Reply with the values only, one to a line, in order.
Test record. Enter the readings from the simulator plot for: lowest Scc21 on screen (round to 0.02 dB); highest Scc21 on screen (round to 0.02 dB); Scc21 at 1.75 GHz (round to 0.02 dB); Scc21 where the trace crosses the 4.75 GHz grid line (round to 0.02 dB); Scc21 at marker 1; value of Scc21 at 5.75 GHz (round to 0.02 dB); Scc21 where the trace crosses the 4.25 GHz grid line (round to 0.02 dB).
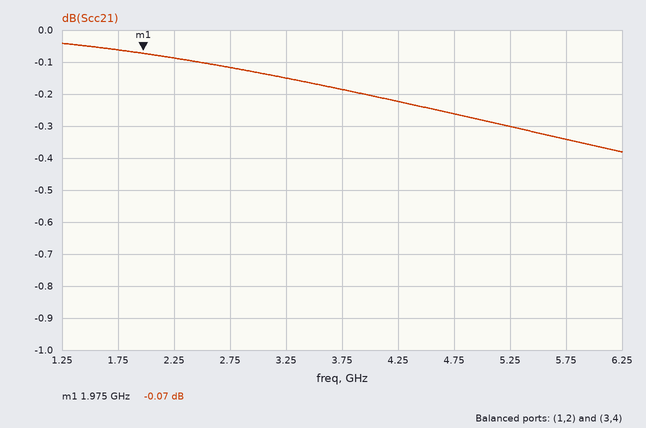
-0.38 dB
-0.04 dB
-0.06 dB
-0.26 dB
-0.07 dB
-0.34 dB
-0.22 dB
